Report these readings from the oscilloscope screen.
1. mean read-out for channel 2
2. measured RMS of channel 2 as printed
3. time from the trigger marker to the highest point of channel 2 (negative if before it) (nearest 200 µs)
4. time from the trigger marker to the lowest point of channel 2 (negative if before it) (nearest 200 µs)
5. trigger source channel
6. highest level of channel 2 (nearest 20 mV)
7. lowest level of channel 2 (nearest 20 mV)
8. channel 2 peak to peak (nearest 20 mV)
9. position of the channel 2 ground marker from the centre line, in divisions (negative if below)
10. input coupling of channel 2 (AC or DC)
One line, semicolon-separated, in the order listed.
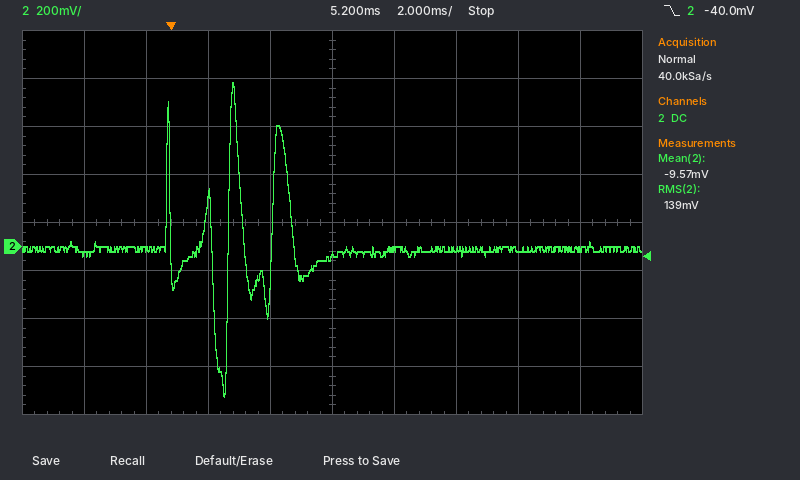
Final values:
-9.57 mV; 139 mV; +2.0 ms; +1.8 ms; channel 2; 680 mV; -620 mV; 1.30 V; -0.5 div; DC
